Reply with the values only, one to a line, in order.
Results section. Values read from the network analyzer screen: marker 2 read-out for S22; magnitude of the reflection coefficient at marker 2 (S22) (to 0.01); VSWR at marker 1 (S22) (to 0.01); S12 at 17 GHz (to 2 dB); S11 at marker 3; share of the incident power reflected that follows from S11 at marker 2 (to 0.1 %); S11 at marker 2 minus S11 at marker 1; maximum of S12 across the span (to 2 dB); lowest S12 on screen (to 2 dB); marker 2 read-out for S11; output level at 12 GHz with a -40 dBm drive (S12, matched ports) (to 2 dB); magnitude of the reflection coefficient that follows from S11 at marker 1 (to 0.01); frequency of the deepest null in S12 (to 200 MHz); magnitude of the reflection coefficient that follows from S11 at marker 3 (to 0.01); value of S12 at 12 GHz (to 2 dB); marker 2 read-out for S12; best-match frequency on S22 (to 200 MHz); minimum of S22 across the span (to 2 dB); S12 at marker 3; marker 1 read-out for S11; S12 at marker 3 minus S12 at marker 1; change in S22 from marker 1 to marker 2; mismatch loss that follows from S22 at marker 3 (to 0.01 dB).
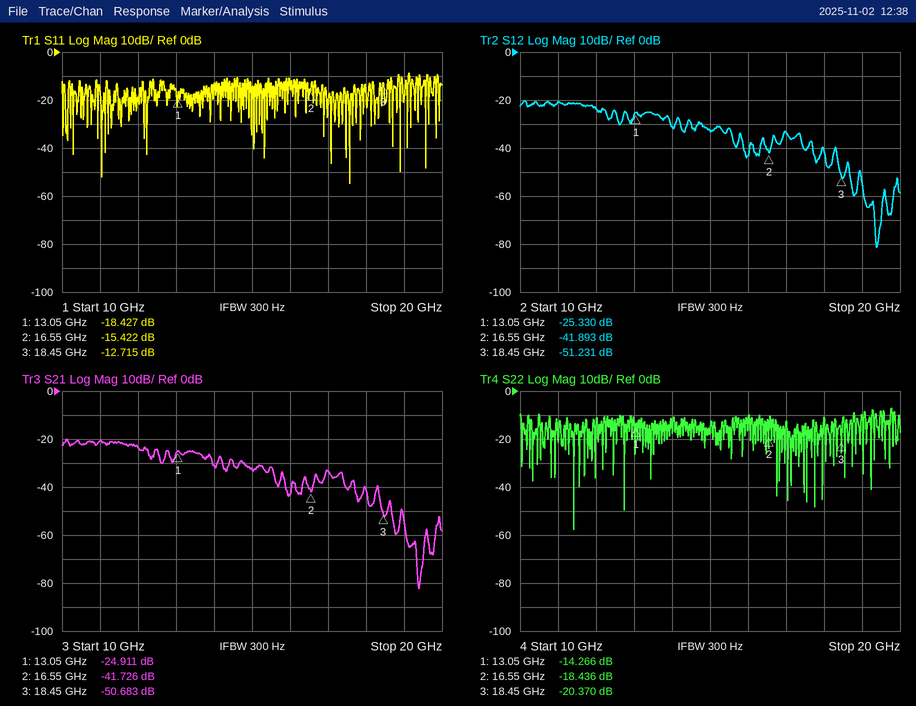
-18.436 dB
0.12
1.48
-34 dB
-12.715 dB
2.9 %
3.005 dB
-20 dB
-82 dB
-15.422 dB
-64 dBm
0.12
19.4 GHz
0.23
-24 dB
-41.893 dB
11.4 GHz
-58 dB
-51.231 dB
-18.427 dB
-25.901 dB
-4.170 dB
0.04 dB
